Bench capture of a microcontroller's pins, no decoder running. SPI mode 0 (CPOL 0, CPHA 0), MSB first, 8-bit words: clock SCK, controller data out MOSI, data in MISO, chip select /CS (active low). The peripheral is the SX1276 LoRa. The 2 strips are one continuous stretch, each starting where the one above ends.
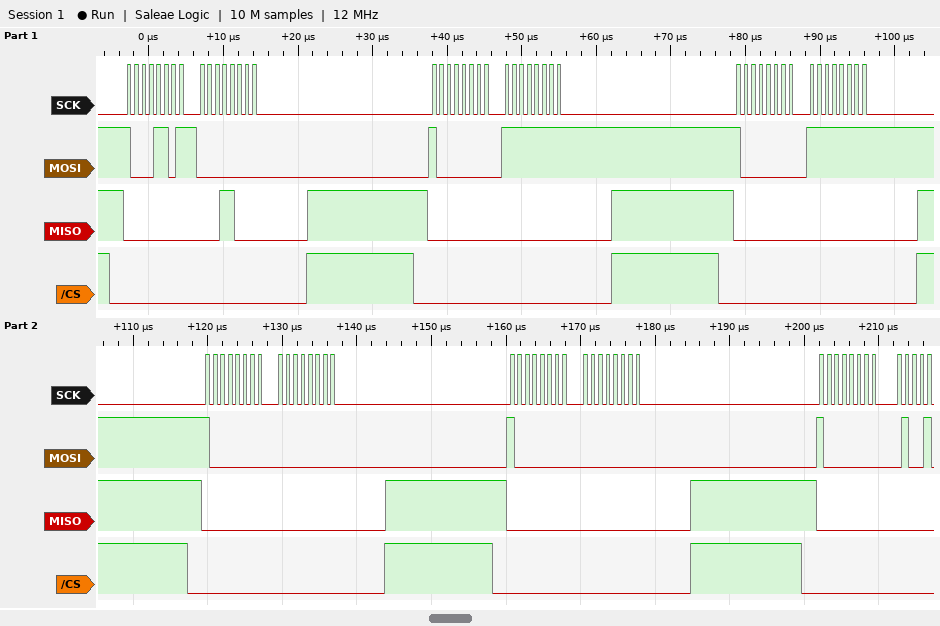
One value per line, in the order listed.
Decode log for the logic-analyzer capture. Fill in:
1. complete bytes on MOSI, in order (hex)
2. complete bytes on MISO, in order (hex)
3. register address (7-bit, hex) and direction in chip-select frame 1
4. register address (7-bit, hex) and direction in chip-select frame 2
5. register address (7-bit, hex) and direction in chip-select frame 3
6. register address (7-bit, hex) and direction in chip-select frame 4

8D 00 80 FF 80 FF 80 00 80 00 80
00 18 00 00 00 00 00 00 00 00 00
0x0D write
0x00 write
0x00 write
0x00 write
